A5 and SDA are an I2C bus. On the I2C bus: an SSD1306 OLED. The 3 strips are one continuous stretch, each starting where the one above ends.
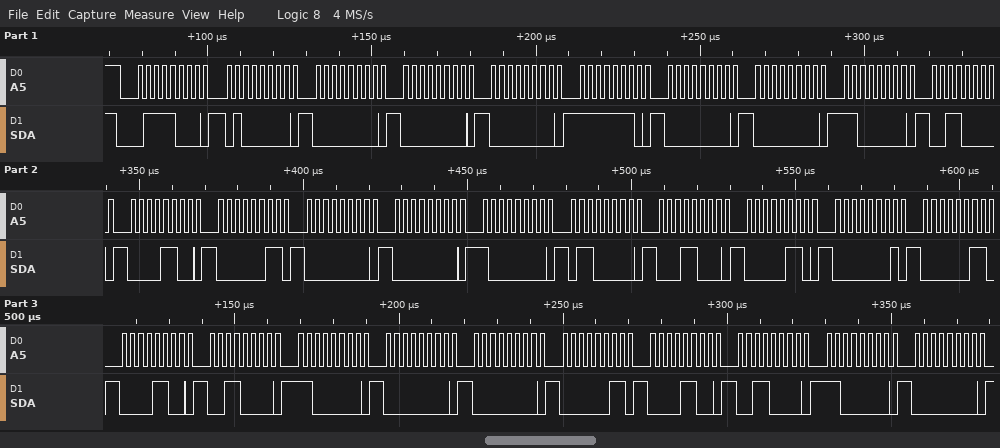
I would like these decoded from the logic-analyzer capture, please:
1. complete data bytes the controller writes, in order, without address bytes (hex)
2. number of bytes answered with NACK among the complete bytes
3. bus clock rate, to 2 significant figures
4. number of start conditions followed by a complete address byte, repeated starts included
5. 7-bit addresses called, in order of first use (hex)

40 00 00 00 FE 00 00 C0 30 0C 03 00 00 80 60 18 06 01 03 0C 30 C0 00 00 03 0C 30 C0 00
0
400 kHz
1
0x3C
